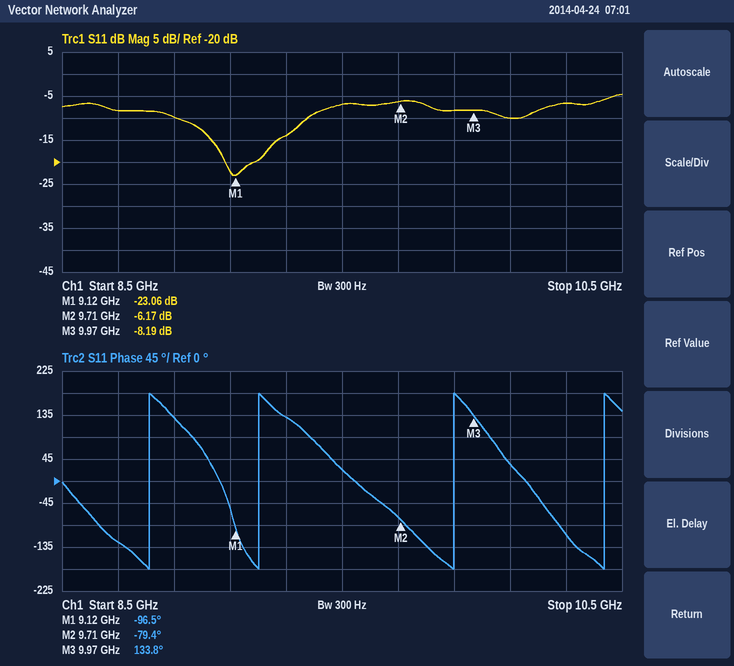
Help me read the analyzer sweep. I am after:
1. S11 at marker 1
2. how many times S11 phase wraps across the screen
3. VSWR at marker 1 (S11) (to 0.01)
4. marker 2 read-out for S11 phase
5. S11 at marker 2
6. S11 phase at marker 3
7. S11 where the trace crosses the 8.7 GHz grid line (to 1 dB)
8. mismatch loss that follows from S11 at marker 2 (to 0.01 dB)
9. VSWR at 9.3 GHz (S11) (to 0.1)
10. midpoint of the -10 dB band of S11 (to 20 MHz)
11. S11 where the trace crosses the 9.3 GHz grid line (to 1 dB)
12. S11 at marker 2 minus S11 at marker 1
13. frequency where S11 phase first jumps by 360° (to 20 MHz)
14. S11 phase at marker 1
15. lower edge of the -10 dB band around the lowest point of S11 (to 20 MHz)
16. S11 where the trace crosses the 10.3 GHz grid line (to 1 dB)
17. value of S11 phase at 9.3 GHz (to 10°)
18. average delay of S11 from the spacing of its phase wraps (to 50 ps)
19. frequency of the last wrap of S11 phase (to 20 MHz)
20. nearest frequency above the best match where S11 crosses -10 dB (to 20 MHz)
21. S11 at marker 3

-23.06 dB
4
1.15
-79.4°
-6.17 dB
133.8°
-8 dB
1.20 dB
1.5
9.14 GHz
-14 dB
16.89 dB
8.82 GHz
-96.5°
8.90 GHz
-7 dB
130°
1.85 ns
10.44 GHz
9.38 GHz
-8.19 dB
